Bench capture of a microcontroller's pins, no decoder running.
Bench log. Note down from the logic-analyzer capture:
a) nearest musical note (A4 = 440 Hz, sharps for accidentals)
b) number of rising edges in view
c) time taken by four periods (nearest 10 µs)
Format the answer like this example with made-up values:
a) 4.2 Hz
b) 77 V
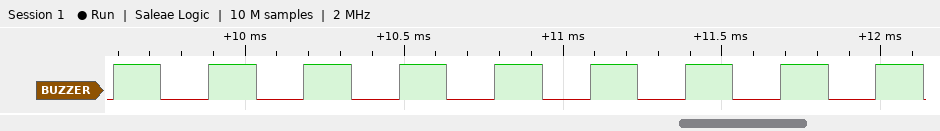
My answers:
a) G#7
b) 9
c) 1200 µs
